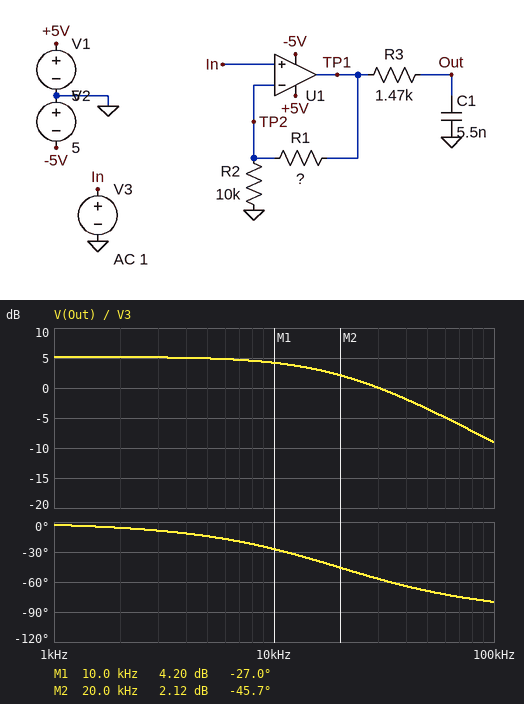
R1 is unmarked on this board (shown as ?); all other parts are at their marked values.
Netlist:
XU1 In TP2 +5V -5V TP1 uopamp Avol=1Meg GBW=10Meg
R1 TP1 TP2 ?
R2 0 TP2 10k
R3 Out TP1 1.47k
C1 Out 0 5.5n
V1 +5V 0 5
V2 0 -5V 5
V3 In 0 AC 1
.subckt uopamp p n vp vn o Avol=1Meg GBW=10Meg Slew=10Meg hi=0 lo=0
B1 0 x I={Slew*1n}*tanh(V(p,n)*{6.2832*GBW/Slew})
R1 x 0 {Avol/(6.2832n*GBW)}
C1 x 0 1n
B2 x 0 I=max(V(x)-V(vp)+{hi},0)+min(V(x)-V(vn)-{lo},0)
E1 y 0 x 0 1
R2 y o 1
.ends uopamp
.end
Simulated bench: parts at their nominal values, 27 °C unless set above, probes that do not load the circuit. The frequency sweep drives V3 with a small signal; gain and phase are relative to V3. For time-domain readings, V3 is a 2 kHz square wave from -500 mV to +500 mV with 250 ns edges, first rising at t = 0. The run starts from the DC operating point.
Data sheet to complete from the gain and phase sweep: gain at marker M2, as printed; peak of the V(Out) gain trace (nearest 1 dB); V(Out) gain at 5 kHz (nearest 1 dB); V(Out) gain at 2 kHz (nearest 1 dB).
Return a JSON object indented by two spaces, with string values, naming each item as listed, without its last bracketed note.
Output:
{
  "gain at marker M2, as printed": "2.12 dB",
  "peak of the V(Out) gain trace": "5 dB",
  "V(Out) gain at 5 kHz": "5 dB",
  "V(Out) gain at 2 kHz": "5 dB"
}
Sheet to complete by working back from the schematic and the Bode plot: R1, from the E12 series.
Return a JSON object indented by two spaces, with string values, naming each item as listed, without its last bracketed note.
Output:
{
  "R1, from the E12 series": "8.2 kΩ"
}
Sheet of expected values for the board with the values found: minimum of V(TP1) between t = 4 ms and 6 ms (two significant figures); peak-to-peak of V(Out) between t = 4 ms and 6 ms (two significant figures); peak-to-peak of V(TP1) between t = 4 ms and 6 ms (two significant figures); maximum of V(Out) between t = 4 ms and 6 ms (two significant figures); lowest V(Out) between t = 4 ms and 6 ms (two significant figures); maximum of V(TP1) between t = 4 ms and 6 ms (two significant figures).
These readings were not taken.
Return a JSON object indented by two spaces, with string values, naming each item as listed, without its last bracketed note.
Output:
{
  "minimum of V(TP1) between t = 4 ms and 6 ms": "-910 mV",
  "peak-to-peak of V(Out) between t = 4 ms and 6 ms": "1.8 V",
  "peak-to-peak of V(TP1) between t = 4 ms and 6 ms": "1.8 V",
  "maximum of V(Out) between t = 4 ms and 6 ms": "910 mV",
  "lowest V(Out) between t = 4 ms and 6 ms": "-910 mV",
  "maximum of V(TP1) between t = 4 ms and 6 ms": "910 mV"
}
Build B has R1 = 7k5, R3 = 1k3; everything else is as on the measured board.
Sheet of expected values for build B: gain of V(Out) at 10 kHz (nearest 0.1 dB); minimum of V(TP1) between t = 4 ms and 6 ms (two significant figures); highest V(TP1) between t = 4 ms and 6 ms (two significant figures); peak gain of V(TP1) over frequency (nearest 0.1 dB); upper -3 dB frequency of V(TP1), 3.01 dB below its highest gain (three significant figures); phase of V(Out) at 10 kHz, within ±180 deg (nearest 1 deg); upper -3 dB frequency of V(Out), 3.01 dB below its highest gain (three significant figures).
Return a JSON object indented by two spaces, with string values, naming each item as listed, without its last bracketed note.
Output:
{
  "gain of V(Out) at 10 kHz": "4.1 dB",
  "minimum of V(TP1) between t = 4 ms and 6 ms": "-880 mV",
  "highest V(TP1) between t = 4 ms and 6 ms": "880 mV",
  "peak gain of V(TP1) over frequency": "4.9 dB",
  "upper -3 dB frequency of V(TP1), 3.01 dB below its highest gain": "5.71 MHz",
  "phase of V(Out) at 10 kHz, within ±180 deg": "-24 deg",
  "upper -3 dB frequency of V(Out), 3.01 dB below its highest gain": "22.3 kHz"
}
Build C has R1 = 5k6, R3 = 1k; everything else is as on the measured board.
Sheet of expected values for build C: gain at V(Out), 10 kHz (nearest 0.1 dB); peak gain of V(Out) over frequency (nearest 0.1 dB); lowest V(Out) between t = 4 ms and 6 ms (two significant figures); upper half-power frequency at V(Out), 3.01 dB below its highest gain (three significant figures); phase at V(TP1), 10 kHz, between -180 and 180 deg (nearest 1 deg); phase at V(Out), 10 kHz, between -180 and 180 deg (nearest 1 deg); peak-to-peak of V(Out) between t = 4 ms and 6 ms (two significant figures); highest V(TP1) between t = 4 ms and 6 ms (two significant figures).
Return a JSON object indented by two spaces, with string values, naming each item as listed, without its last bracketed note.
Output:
{
  "gain at V(Out), 10 kHz": "3.4 dB",
  "peak gain of V(Out) over frequency": "3.9 dB",
  "lowest V(Out) between t = 4 ms and 6 ms": "-780 mV",
  "upper half-power frequency at V(Out), 3.01 dB below its highest gain": "28.9 kHz",
  "phase at V(TP1), 10 kHz, between -180 and 180 deg": "0 deg",
  "phase at V(Out), 10 kHz, between -180 and 180 deg": "-19 deg",
  "peak-to-peak of V(Out) between t = 4 ms and 6 ms": "1.6 V",
  "highest V(TP1) between t = 4 ms and 6 ms": "780 mV"
}
